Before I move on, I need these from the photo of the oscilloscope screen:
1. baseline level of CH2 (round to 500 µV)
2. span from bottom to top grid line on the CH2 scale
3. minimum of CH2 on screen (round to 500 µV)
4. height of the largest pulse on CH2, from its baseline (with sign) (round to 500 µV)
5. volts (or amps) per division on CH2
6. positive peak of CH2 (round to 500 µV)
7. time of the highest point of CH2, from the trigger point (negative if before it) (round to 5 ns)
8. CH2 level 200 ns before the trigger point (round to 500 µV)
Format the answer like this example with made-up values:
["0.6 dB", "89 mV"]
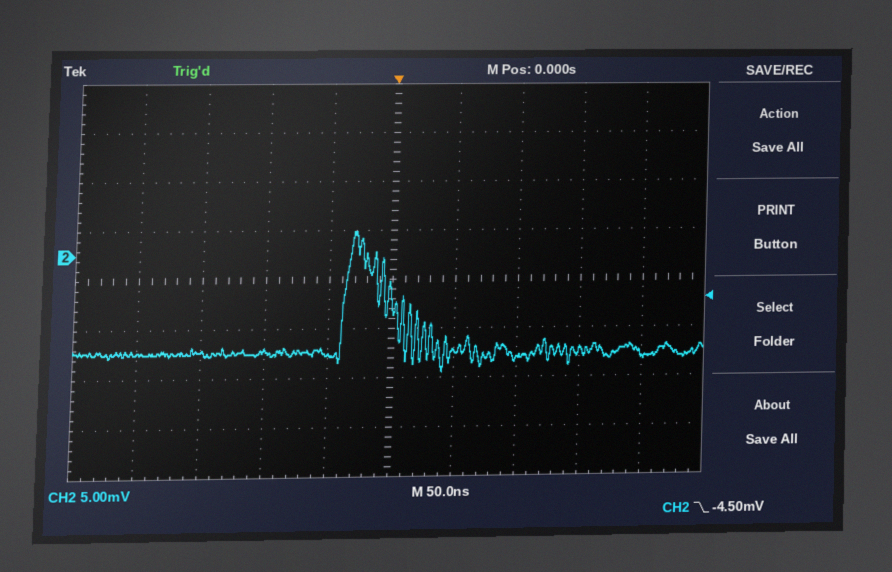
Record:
["-10.0 mV", "40 mV", "-12.0 mV", "+12.5 mV", "5 mV", "2.5 mV", "-30 ns", "-10.0 mV"]
